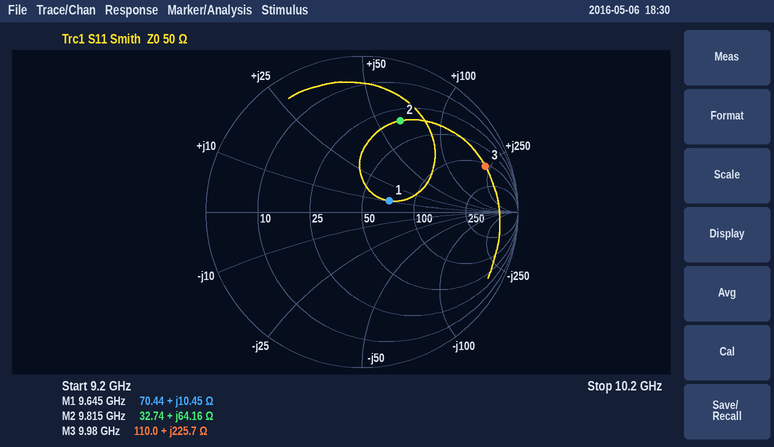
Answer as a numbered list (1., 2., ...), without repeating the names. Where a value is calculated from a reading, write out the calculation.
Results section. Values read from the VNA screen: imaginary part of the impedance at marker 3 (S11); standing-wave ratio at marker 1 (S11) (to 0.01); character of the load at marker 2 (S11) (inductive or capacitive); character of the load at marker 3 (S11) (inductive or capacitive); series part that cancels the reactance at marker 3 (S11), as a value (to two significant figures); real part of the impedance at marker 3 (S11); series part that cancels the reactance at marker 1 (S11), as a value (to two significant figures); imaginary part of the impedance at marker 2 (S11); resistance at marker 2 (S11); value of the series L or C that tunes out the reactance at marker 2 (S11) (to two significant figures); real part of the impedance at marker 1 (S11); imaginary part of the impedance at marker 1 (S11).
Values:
1. +225.7 Ω
2. 1.47
3. inductive
4. inductive
5. C = 1/(2π × 9.98 GHz × 225.7 Ω) ≈ 71 fF
6. 110.0 Ω
7. C = 1/(2π × 9.645 GHz × 10.45 Ω) ≈ 1.6 pF
8. +64.16 Ω
9. 32.74 Ω
10. C = 1/(2π × 9.815 GHz × 64.16 Ω) ≈ 253 fF, so 250 fF to two significant figures
11. 70.44 Ω
12. +10.45 Ω
